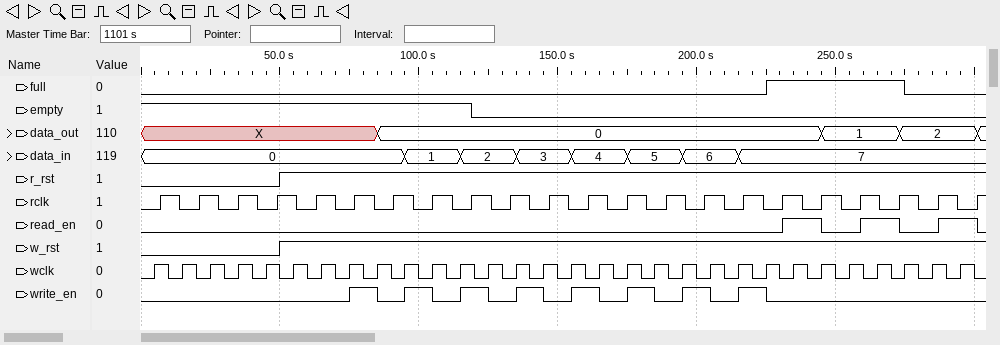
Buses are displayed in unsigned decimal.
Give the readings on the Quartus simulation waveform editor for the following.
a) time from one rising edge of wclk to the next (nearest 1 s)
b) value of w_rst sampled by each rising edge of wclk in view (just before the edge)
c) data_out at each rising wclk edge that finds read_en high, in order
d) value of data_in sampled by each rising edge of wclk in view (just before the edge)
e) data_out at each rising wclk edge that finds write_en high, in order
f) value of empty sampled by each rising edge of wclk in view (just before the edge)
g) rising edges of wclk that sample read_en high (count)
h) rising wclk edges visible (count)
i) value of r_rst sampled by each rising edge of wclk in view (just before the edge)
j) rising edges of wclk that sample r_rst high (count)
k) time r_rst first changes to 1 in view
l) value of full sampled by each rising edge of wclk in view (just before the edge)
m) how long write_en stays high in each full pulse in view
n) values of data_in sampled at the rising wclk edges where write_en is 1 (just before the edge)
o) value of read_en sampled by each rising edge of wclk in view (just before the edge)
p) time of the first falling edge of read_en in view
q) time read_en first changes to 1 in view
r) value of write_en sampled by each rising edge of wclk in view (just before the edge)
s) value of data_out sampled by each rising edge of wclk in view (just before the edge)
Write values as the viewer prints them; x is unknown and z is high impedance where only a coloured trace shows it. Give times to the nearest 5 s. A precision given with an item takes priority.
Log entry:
10 s
0 0 0 0 0 1 1 1 1 1 1 1 1 1 1 1 1 1 1 1 1 1 1 1 1 1 1 1 1 1
0, 0, 1, 2
0, 0, 0, 0, 0, 0, 0, 0, 0, 0, 1, 1, 2, 2, 3, 3, 4, 4, 5, 5, 6, 6, 7, 7, 7, 7, 7, 7, 7, 7
X, 0, 0, 0, 0, 0, 0, 0
1 1 1 1 1 1 1 1 1 1 1 1 0 0 0 0 0 0 0 0 0 0 0 0 0 0 0 0 0 0
4
30
0 0 0 0 0 1 1 1 1 1 1 1 1 1 1 1 1 1 1 1 1 1 1 1 1 1 1 1 1 1
25
50 s
0 0 0 0 0 0 0 0 0 0 0 0 0 0 0 0 0 0 0 0 0 0 0 1 1 1 1 1 0 0
10 s, 10 s, 10 s, 10 s, 10 s, 10 s, 10 s, 10 s
0, 1, 2, 3, 4, 5, 6, 7
0 0 0 0 0 0 0 0 0 0 0 0 0 0 0 0 0 0 0 0 0 0 0 1 1 0 1 0 0 1
245 s
230 s
0 0 0 0 0 0 0 0 1 0 1 0 1 0 1 0 1 0 1 0 1 0 1 0 0 0 0 0 0 0
X, X, X, X, X, X, X, X, X, 0, 0, 0, 0, 0, 0, 0, 0, 0, 0, 0, 0, 0, 0, 0, 0, 1, 1, 2, 2, 2
